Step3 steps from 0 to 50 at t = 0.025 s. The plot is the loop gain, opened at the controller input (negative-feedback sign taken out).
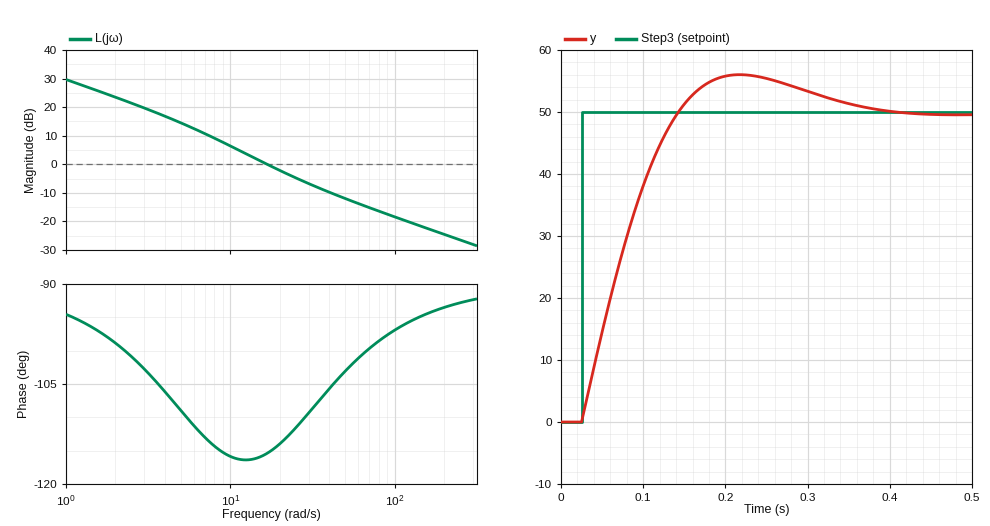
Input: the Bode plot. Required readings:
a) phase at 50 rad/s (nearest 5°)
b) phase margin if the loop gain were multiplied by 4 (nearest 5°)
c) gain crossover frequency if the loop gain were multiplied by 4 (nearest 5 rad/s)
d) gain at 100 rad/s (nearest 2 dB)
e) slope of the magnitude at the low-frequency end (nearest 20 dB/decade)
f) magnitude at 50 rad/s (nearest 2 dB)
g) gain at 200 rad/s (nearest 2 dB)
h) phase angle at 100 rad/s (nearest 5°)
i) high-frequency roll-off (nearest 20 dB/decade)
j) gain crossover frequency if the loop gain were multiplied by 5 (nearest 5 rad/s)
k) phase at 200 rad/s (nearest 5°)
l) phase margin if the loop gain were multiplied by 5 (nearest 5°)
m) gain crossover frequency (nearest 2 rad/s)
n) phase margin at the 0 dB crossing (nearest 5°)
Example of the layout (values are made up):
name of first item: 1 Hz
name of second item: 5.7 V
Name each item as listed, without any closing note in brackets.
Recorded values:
phase at 50 rad/s: -105°
phase margin if the loop gain were multiplied by 4: 75°
gain crossover frequency if the loop gain were multiplied by 4: 50 rad/s
gain at 100 rad/s: -18 dB
slope of the magnitude at the low-frequency end: -20 dB/decade
magnitude at 50 rad/s: -12 dB
gain at 200 rad/s: -24 dB
phase angle at 100 rad/s: -95°
high-frequency roll-off: -20 dB/decade
gain crossover frequency if the loop gain were multiplied by 5: 60 rad/s
phase at 200 rad/s: -95°
phase margin if the loop gain were multiplied by 5: 80°
gain crossover frequency: 16 rad/s
phase margin at the 0 dB crossing: 65°
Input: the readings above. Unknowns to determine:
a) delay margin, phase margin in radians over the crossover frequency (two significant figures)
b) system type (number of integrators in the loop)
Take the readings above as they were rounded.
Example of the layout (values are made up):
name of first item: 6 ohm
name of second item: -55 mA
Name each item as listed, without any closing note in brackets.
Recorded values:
delay margin, phase margin in radians over the crossover frequency: 0.071 s
system type: 1
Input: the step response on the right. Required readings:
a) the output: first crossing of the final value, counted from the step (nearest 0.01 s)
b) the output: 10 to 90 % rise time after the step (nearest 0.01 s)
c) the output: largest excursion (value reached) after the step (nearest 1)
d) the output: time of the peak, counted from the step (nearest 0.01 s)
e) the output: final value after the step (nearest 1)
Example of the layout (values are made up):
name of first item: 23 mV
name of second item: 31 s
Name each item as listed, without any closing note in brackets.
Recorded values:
the output: first crossing of the final value, counted from the step: 0.12 s
the output: 10 to 90 % rise time after the step: 0.09 s
the output: largest excursion (value reached) after the step: 56
the output: time of the peak, counted from the step: 0.19 s
the output: final value after the step: 50
